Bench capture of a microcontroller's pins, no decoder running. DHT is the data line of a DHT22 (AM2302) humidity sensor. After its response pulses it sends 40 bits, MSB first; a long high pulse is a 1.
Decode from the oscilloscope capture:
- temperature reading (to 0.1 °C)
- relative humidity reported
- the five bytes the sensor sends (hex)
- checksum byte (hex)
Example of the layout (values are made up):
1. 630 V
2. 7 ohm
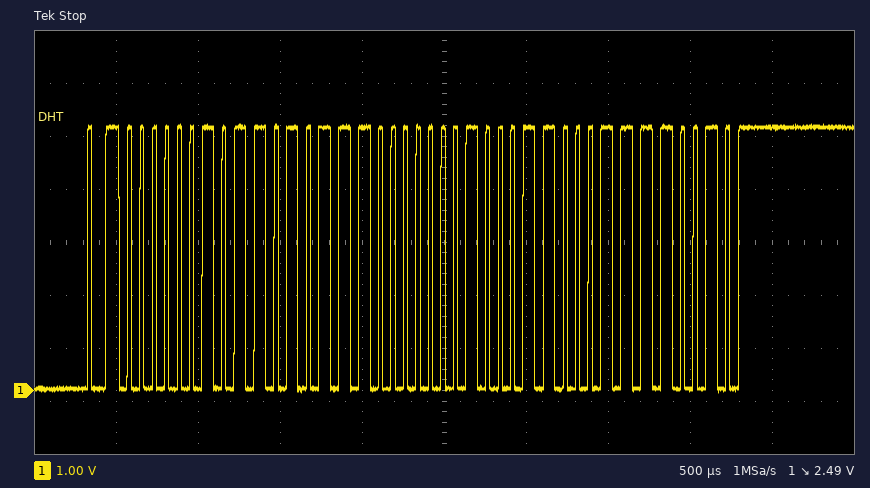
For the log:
1. 28.0 °C
2. 72.7 %
3. 02 D7 01 18 F2
4. 0xF2
